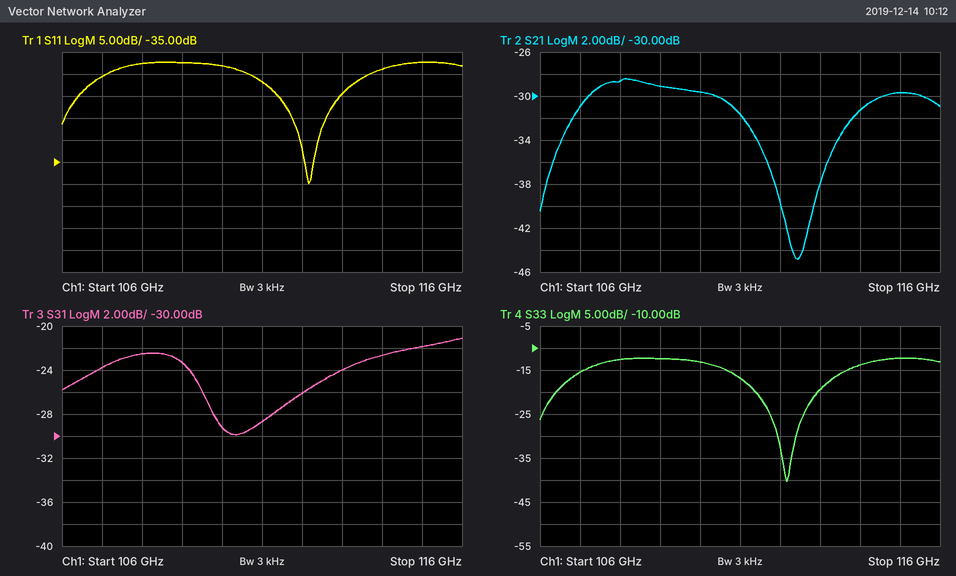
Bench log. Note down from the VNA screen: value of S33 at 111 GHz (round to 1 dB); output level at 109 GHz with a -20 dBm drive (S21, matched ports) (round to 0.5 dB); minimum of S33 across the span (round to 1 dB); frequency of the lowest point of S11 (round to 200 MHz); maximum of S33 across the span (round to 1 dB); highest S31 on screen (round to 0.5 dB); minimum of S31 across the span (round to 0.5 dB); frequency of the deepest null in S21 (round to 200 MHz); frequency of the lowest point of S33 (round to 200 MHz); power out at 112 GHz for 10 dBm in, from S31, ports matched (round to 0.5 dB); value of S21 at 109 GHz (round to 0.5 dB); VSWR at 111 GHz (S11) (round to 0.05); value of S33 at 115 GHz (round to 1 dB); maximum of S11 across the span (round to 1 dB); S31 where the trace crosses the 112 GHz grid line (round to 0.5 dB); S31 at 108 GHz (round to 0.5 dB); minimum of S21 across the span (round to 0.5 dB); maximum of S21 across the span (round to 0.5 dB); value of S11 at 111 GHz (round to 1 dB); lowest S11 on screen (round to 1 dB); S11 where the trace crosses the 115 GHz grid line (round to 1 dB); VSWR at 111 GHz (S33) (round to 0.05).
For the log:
-17 dB
-49.0 dBm
-40 dB
112.2 GHz
-12 dB
-21.0 dB
-30.0 dB
112.4 GHz
112.2 GHz
-16.0 dBm
-29.0 dB
1.35
-12 dB
-12 dB
-26.0 dB
-22.5 dB
-45.0 dB
-28.5 dB
-17 dB
-40 dB
-12 dB
1.35
